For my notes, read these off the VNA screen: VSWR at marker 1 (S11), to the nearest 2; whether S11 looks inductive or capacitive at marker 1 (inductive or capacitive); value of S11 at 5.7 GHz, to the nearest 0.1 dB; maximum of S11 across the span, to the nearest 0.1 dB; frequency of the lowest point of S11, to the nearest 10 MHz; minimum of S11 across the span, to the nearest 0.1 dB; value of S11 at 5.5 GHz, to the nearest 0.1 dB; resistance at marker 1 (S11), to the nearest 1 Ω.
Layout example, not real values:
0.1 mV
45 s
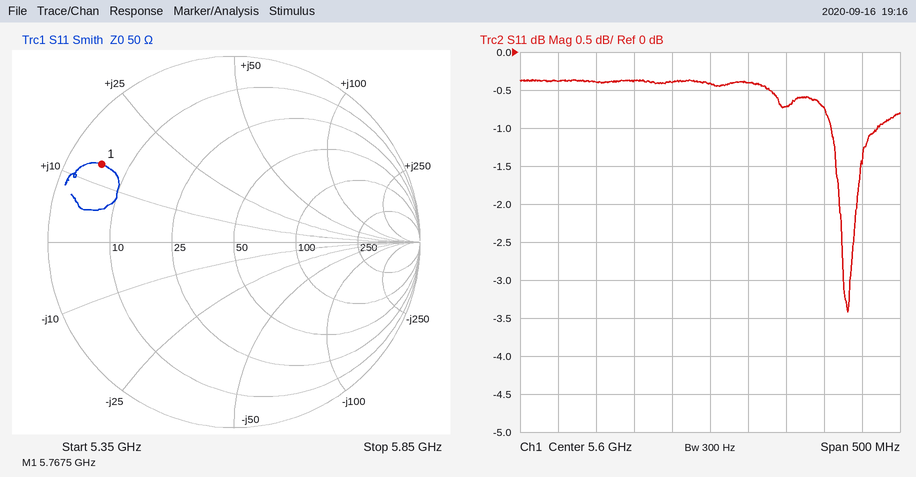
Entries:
10
inductive
-0.7 dB
-0.4 dB
5.78 GHz
-3.4 dB
-0.4 dB
5 Ω
